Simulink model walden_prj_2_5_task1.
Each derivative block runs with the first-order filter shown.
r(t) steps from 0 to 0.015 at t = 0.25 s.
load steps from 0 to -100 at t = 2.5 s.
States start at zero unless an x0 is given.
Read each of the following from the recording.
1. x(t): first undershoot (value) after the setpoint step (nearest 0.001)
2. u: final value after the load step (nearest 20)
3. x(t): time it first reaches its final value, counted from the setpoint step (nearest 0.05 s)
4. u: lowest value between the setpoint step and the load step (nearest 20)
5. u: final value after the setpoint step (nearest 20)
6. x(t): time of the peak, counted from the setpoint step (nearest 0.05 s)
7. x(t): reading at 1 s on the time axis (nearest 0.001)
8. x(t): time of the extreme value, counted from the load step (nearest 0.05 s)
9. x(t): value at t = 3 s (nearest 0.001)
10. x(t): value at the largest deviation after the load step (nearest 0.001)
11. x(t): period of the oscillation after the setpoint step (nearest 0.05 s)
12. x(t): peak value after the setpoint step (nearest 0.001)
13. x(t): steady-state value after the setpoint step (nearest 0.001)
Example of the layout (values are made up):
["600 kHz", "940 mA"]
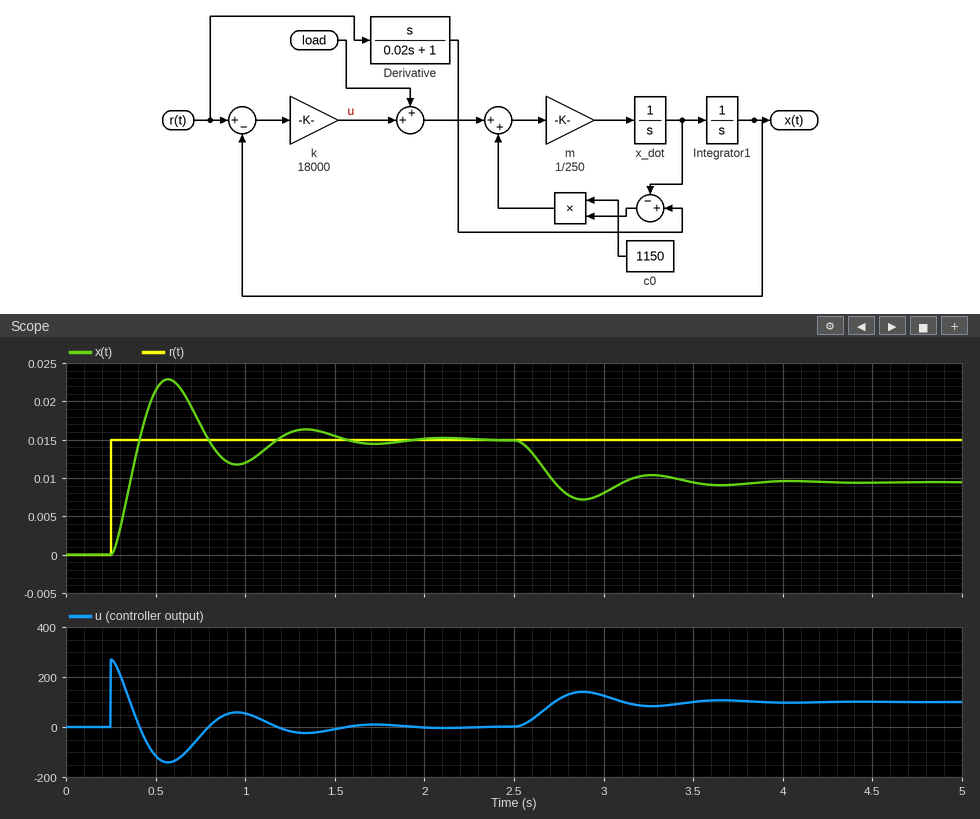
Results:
["0.012", "100", "0.15 s", "-140", "0", "0.30 s", "0.012", "0.40 s", "0.008", "0.007", "0.75 s", "0.023", "0.015"]
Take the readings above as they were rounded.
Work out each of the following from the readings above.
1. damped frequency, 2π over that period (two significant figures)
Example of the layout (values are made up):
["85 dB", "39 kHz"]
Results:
["8.4 rad/s"]
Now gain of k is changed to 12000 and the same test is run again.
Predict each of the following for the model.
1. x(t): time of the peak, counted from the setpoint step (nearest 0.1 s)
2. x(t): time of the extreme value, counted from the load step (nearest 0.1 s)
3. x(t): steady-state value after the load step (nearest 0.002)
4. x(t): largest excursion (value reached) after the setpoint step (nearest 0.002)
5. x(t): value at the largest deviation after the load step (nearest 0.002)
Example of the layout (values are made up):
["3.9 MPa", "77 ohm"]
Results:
["0.4 s", "0.5 s", "0.006", "0.022", "0.004"]
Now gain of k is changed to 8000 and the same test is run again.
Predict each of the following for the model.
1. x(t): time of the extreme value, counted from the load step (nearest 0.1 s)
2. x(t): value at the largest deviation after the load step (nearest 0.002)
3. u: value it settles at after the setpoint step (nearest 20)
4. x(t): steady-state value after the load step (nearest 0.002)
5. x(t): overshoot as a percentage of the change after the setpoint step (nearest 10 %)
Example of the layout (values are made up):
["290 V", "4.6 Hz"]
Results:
["0.6 s", "0.000", "0", "0.002", "40 %"]
